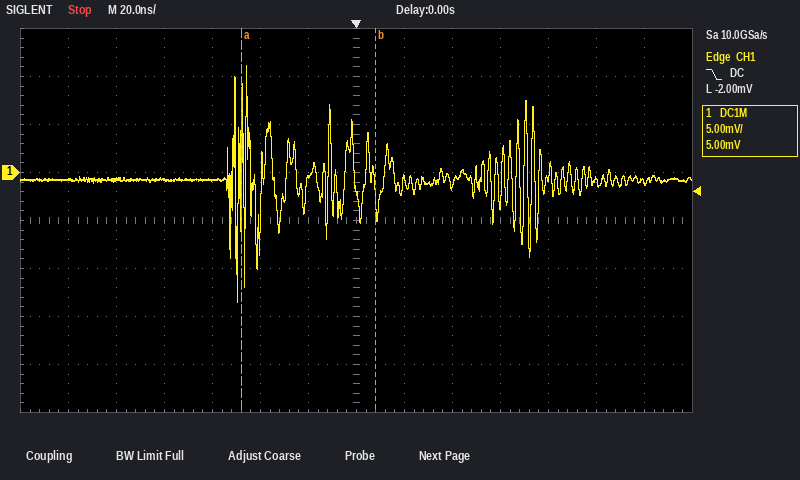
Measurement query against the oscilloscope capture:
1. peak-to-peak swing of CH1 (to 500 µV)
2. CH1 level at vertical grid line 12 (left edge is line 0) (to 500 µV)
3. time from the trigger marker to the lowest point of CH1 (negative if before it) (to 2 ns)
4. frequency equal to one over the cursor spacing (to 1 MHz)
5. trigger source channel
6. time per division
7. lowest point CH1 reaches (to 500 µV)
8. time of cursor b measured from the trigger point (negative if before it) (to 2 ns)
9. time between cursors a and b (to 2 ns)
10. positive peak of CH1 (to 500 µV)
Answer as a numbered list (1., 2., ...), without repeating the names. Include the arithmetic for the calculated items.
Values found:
1. 11.0 mV − (-13.5 mV) = 24.5 mV
2. -1.0 mV
3. -50 ns
4. 1 / 56 ns ≈ 18 MHz
5. CH1
6. 20 ns
7. -13.5 mV
8. +8 ns
9. 56 ns
10. 11.0 mV
